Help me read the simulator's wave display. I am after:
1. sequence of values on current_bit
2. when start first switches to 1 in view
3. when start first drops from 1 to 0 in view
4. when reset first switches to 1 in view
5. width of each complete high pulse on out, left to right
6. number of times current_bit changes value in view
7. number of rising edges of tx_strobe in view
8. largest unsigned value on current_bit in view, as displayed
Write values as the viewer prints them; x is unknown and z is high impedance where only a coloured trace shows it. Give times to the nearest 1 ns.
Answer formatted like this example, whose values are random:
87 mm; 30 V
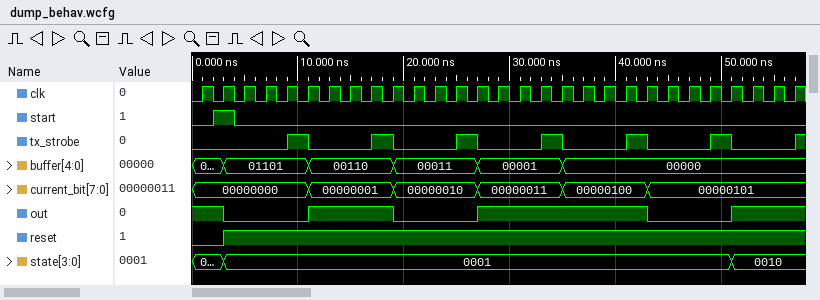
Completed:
00000000, 00000001, 00000010, 00000011, 00000100, 00000101; 2 ns; 4 ns; 3 ns; 8 ns, 16 ns; 5; 7; 00000101
